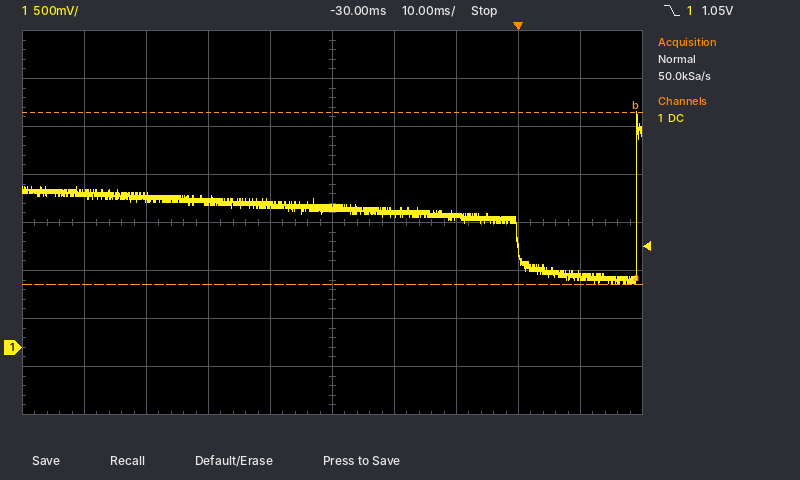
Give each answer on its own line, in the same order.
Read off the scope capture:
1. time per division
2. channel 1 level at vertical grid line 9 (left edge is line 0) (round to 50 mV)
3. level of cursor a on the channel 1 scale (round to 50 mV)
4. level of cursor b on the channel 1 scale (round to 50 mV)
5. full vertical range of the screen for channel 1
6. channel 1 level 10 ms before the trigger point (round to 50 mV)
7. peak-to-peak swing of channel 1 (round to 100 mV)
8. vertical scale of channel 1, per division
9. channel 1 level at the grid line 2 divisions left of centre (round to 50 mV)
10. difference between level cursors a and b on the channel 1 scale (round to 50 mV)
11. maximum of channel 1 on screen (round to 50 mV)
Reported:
10 ms
750 mV
650 mV
2.45 V
4 V
1.35 V
1.80 V
500 mV
1.50 V
1.80 V
2.45 V
